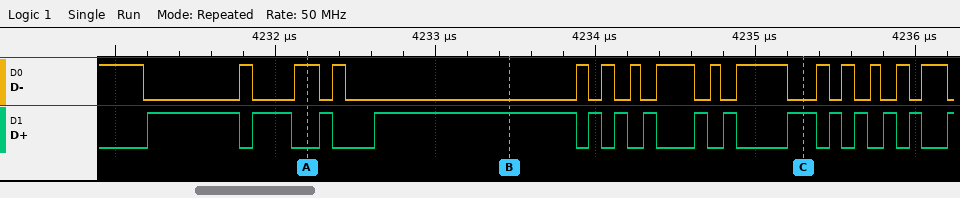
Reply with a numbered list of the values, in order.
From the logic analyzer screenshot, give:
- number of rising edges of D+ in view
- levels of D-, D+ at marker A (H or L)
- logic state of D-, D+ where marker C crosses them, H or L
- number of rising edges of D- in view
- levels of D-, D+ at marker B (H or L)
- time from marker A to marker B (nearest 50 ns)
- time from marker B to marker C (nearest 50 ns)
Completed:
1. 15
2. D-=H, D+=L
3. D-=L, D+=H
4. 14
5. D-=L, D+=H
6. 1250 ns
7. 1850 ns
